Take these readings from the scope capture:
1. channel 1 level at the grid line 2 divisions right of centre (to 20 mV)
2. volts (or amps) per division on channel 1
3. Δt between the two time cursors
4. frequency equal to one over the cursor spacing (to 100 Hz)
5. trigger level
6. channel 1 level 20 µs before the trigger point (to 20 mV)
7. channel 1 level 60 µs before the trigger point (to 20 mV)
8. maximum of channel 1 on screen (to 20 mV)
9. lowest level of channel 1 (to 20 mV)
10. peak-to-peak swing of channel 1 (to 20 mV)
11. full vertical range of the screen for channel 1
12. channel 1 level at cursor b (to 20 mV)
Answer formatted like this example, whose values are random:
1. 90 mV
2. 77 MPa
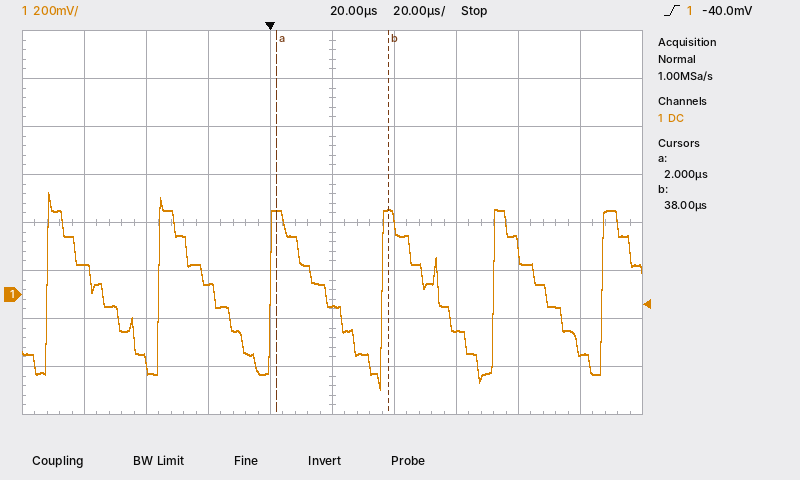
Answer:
1. -160 mV
2. 200 mV
3. 36 µs
4. 27.8 kHz
5. -40.0 mV
6. 40 mV
7. 120 mV
8. 420 mV
9. -400 mV
10. 820 mV
11. 1.6 V
12. 360 mV
